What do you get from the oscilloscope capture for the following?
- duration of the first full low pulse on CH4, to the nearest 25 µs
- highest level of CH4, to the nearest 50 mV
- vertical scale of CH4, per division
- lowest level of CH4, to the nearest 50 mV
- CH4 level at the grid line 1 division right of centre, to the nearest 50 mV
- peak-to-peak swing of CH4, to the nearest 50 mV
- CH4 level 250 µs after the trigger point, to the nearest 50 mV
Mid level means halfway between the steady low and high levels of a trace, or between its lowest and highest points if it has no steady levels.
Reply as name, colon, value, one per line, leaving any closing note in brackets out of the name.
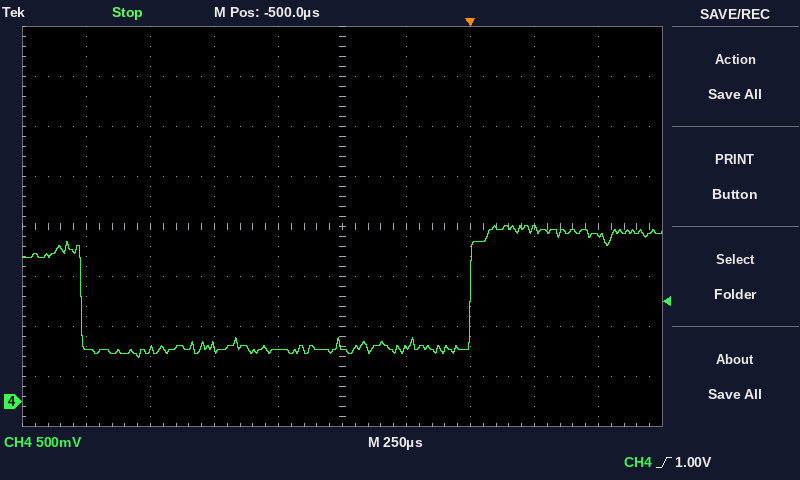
duration of the first full low pulse on CH4, to the nearest 25 µs: 1.525 ms
highest level of CH4, to the nearest 50 mV: 1.75 V
vertical scale of CH4, per division: 500 mV
lowest level of CH4, to the nearest 50 mV: 450 mV
CH4 level at the grid line 1 division right of centre, to the nearest 50 mV: 550 mV
peak-to-peak swing of CH4, to the nearest 50 mV: 1.30 V
CH4 level 250 µs after the trigger point, to the nearest 50 mV: 1.75 V
